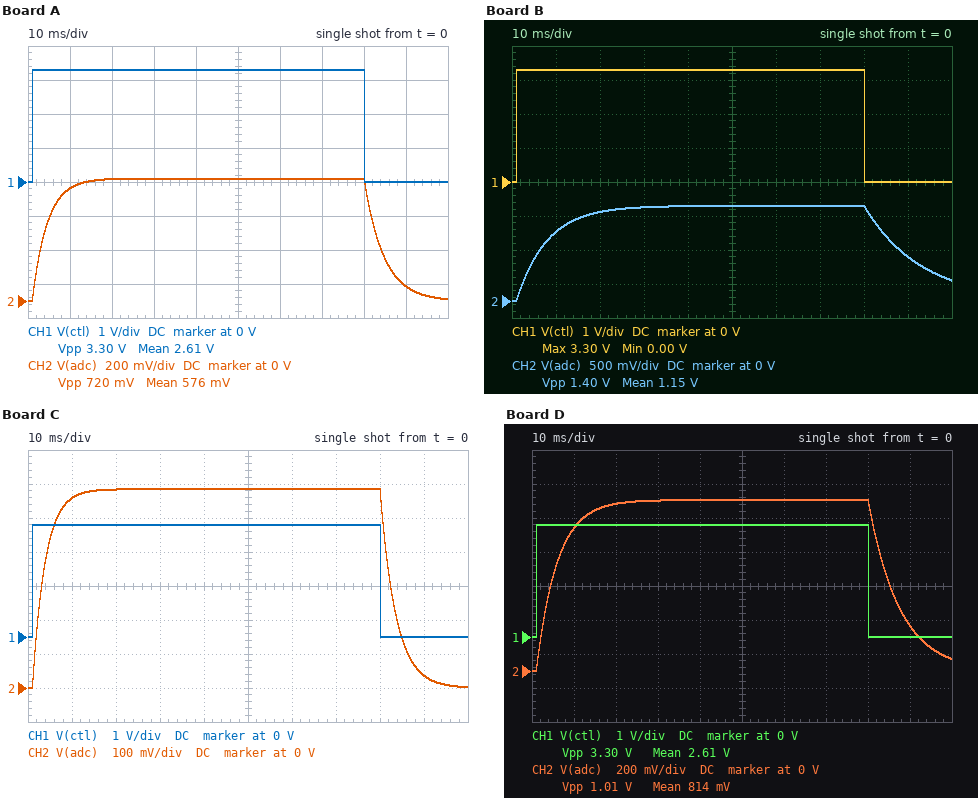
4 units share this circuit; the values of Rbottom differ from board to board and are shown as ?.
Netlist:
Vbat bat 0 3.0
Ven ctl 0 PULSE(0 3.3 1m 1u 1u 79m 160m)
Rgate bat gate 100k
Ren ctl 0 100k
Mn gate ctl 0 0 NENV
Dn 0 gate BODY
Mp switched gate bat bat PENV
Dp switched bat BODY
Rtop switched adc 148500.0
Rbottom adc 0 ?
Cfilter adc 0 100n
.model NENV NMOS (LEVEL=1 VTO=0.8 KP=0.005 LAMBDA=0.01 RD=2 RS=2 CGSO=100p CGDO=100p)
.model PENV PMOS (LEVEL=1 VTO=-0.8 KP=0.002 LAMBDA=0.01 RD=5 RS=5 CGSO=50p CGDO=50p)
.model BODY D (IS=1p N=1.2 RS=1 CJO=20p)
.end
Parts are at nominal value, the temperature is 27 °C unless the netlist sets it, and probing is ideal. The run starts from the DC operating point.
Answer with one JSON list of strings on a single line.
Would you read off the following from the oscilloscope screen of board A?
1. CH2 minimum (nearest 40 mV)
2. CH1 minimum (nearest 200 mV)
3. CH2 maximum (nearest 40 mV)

["0 V", "0 V", "720 mV"]
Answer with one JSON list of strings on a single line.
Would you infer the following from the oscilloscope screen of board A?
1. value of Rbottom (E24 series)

["47 kΩ"]
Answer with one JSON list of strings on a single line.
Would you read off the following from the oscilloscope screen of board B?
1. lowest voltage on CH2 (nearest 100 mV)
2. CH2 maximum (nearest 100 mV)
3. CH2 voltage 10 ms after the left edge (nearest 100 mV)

["0 V", "1.4 V", "1.0 V"]
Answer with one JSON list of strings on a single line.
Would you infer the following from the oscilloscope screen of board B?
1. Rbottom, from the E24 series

["130 kΩ"]
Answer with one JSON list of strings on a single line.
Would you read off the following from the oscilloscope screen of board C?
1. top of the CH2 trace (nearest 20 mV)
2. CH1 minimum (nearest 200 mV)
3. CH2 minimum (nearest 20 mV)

["580 mV", "0 V", "0 V"]
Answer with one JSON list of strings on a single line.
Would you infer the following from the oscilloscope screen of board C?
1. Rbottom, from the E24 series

["36 kΩ"]
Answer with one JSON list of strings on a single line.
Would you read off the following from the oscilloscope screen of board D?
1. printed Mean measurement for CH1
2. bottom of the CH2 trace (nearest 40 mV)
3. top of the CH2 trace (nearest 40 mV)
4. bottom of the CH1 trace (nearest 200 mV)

["2.61 V", "0 V", "1.00 V", "0 V"]
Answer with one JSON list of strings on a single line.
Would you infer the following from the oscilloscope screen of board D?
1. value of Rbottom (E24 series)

["75 kΩ"]
